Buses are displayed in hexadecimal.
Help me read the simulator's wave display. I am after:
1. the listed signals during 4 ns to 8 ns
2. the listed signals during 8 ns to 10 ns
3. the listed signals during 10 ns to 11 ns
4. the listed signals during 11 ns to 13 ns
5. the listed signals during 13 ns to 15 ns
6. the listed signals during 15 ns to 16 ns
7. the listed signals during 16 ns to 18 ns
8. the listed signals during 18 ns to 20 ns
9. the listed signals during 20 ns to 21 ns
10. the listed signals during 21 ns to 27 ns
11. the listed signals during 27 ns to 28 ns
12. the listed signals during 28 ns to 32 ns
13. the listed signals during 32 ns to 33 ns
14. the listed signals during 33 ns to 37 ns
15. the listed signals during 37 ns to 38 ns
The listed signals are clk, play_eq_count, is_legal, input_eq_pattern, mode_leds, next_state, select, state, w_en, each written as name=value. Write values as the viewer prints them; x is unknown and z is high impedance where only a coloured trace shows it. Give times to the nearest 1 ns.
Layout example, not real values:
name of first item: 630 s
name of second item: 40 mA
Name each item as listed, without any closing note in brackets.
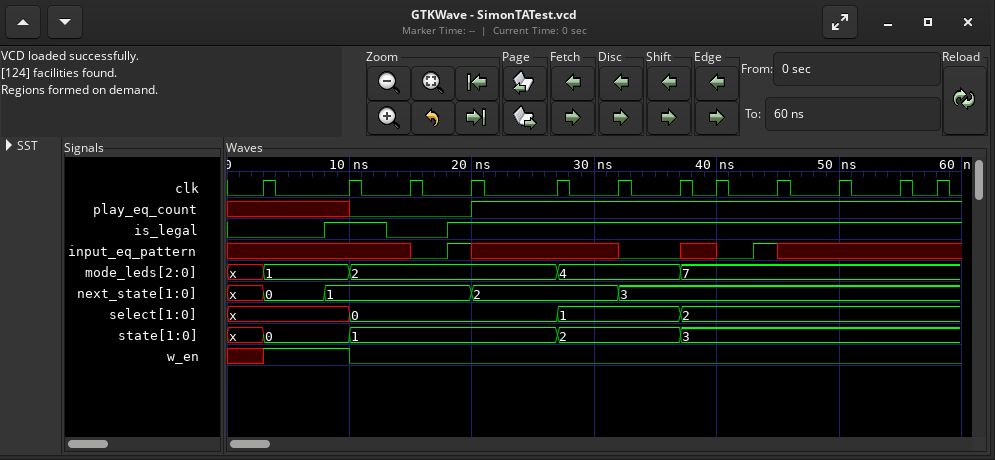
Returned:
the listed signals during 4 ns to 8 ns: clk=0, play_eq_count=x, is_legal=0, input_eq_pattern=x, mode_leds=1, next_state=0, select=x, state=0, w_en=1
the listed signals during 8 ns to 10 ns: clk=0, play_eq_count=x, is_legal=1, input_eq_pattern=x, mode_leds=1, next_state=1, select=x, state=0, w_en=1
the listed signals during 10 ns to 11 ns: clk=1, play_eq_count=0, is_legal=1, input_eq_pattern=x, mode_leds=2, next_state=1, select=0, state=1, w_en=0
the listed signals during 11 ns to 13 ns: clk=0, play_eq_count=0, is_legal=1, input_eq_pattern=x, mode_leds=2, next_state=1, select=0, state=1, w_en=0
the listed signals during 13 ns to 15 ns: clk=0, play_eq_count=0, is_legal=0, input_eq_pattern=x, mode_leds=2, next_state=1, select=0, state=1, w_en=0
the listed signals during 15 ns to 16 ns: clk=1, play_eq_count=0, is_legal=0, input_eq_pattern=0, mode_leds=2, next_state=1, select=0, state=1, w_en=0
the listed signals during 16 ns to 18 ns: clk=0, play_eq_count=0, is_legal=0, input_eq_pattern=0, mode_leds=2, next_state=1, select=0, state=1, w_en=0
the listed signals during 18 ns to 20 ns: clk=0, play_eq_count=0, is_legal=1, input_eq_pattern=1, mode_leds=2, next_state=1, select=0, state=1, w_en=0
the listed signals during 20 ns to 21 ns: clk=1, play_eq_count=1, is_legal=1, input_eq_pattern=x, mode_leds=2, next_state=2, select=0, state=1, w_en=0
the listed signals during 21 ns to 27 ns: clk=0, play_eq_count=1, is_legal=1, input_eq_pattern=x, mode_leds=2, next_state=2, select=0, state=1, w_en=0
the listed signals during 27 ns to 28 ns: clk=1, play_eq_count=1, is_legal=1, input_eq_pattern=x, mode_leds=4, next_state=2, select=1, state=2, w_en=0
the listed signals during 28 ns to 32 ns: clk=0, play_eq_count=1, is_legal=1, input_eq_pattern=x, mode_leds=4, next_state=2, select=1, state=2, w_en=0
the listed signals during 32 ns to 33 ns: clk=1, play_eq_count=1, is_legal=1, input_eq_pattern=0, mode_leds=4, next_state=3, select=1, state=2, w_en=0
the listed signals during 33 ns to 37 ns: clk=0, play_eq_count=1, is_legal=1, input_eq_pattern=0, mode_leds=4, next_state=3, select=1, state=2, w_en=0
the listed signals during 37 ns to 38 ns: clk=1, play_eq_count=1, is_legal=1, input_eq_pattern=x, mode_leds=7, next_state=3, select=2, state=3, w_en=0
